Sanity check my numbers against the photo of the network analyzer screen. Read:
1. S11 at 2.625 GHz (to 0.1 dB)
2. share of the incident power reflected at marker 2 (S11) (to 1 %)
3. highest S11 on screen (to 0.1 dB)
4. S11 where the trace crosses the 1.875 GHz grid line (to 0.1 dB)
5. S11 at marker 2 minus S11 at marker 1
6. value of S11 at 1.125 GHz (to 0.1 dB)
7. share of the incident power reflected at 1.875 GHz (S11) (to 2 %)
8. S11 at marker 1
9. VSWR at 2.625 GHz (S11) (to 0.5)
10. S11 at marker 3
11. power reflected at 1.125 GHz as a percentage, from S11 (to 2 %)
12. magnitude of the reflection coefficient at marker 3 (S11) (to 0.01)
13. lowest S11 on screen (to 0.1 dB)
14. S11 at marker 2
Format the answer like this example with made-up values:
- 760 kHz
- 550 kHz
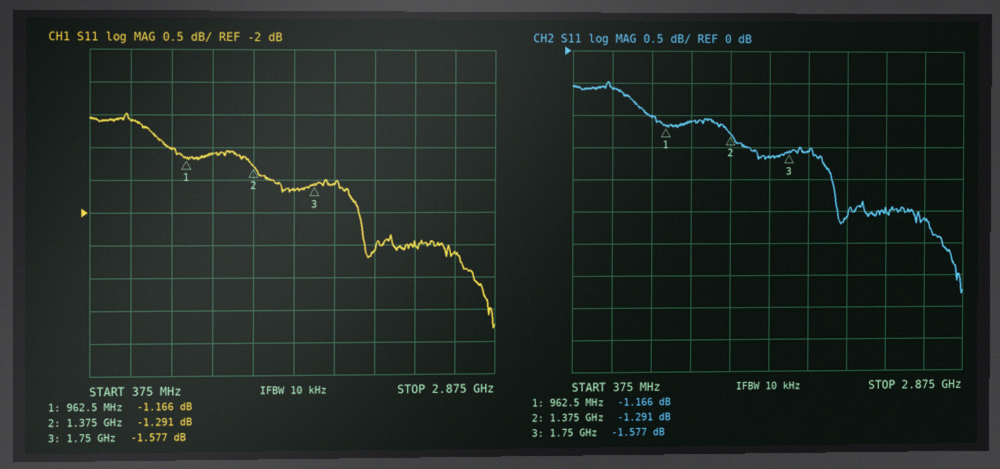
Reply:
- -2.6 dB
- 74 %
- -0.5 dB
- -1.6 dB
- -0.125 dB
- -1.1 dB
- 70 %
- -1.166 dB
- 6.5
- -1.577 dB
- 78 %
- 0.83
- -3.8 dB
- -1.291 dB
